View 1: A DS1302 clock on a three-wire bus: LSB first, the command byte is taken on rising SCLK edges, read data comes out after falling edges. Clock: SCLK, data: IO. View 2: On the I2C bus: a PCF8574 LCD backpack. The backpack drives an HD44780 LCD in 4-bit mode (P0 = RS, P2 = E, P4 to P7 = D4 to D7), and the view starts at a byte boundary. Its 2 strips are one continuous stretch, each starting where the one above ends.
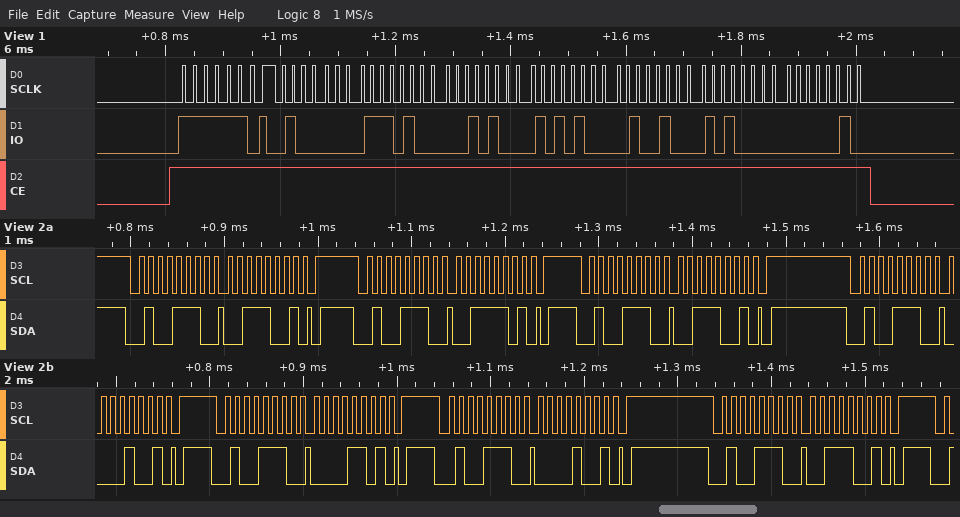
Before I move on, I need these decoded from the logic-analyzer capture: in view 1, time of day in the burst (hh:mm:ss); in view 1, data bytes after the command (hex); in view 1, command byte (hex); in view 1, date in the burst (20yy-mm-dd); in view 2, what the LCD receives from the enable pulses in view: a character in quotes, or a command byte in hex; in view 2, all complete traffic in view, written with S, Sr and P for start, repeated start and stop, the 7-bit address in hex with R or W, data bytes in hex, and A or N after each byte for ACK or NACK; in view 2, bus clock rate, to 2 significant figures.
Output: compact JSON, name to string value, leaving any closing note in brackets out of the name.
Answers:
{"in view 1, time of day in the burst": "14:17:02", "in view 1, data bytes after the command": "02 17 14 15 12 05 20", "in view 1, command byte": "0xBF", "in view 1, date in the burst": "2020-12-15", "in view 2, what the LCD receives from the enable pulses in view: a character in quotes, or a command byte in hex": "'0'", "in view 2, all complete traffic in view, written with S, Sr and P for start, repeated start and stop, the 7-bit address in hex with R or W, data bytes in hex, and A or N after each byte for ACK or NACK": "S 27W A 39 A P S 27W A 3D A P S 27W A 39 A P S 27W A 09 A P S 27W A 0D A P S 27W A 09 A P S 27W A 39 A P", "in view 2, bus clock rate, to 2 significant figures": "100 kHz"}
